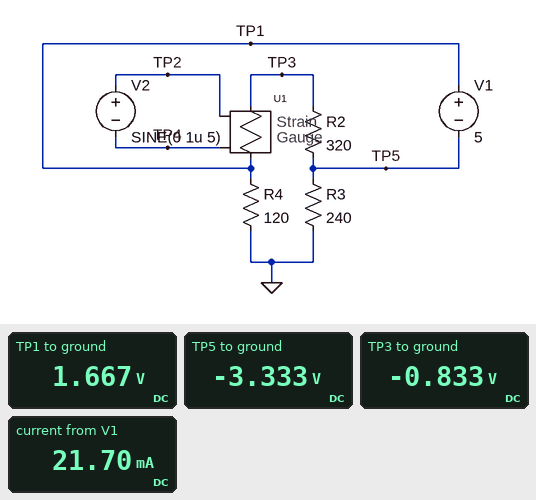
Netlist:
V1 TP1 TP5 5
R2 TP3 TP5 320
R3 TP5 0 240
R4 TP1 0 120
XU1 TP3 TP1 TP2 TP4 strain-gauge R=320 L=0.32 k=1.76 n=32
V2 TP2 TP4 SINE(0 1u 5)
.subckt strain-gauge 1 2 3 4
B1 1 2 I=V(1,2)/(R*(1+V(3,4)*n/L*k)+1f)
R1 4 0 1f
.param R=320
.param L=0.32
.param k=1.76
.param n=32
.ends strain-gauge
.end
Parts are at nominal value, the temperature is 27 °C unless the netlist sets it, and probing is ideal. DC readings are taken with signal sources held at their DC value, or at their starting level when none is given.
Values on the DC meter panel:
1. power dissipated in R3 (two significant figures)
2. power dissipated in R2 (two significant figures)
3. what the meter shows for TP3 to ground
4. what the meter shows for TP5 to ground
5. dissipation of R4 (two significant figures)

46 mW
20 mW
-0.833 V
-3.333 V
23 mW
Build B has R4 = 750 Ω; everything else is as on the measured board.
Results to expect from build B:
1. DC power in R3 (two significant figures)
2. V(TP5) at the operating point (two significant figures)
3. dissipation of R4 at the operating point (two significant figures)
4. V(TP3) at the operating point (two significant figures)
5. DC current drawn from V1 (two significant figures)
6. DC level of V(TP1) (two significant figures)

6.1 mW
-1.2 V
19 mW
1.3 V
13 mA
3.8 V
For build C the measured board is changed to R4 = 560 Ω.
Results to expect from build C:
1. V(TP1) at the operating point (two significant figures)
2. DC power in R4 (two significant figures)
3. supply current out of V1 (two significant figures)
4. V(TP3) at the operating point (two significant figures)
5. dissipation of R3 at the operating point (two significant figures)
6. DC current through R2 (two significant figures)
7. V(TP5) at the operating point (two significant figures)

3.5 V
22 mW
14 mA
1.0 V
9.4 mW
7.8 mA
-1.5 V
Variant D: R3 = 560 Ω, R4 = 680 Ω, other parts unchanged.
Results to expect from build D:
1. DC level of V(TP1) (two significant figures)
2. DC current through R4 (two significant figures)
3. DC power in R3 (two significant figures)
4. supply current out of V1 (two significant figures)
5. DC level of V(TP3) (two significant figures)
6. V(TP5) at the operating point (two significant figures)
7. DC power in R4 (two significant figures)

2.7 V
4.0 mA
9.1 mW
12 mA
240 mV
-2.3 V
11 mW
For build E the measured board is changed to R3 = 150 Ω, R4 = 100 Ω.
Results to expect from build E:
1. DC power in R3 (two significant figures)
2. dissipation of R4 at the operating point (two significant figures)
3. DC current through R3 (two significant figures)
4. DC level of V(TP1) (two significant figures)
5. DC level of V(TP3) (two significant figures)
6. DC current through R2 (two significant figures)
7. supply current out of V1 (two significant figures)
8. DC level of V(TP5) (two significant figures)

60 mW
40 mW
20 mA
2.0 V
-500 mV
7.8 mA
28 mA
-3.0 V
